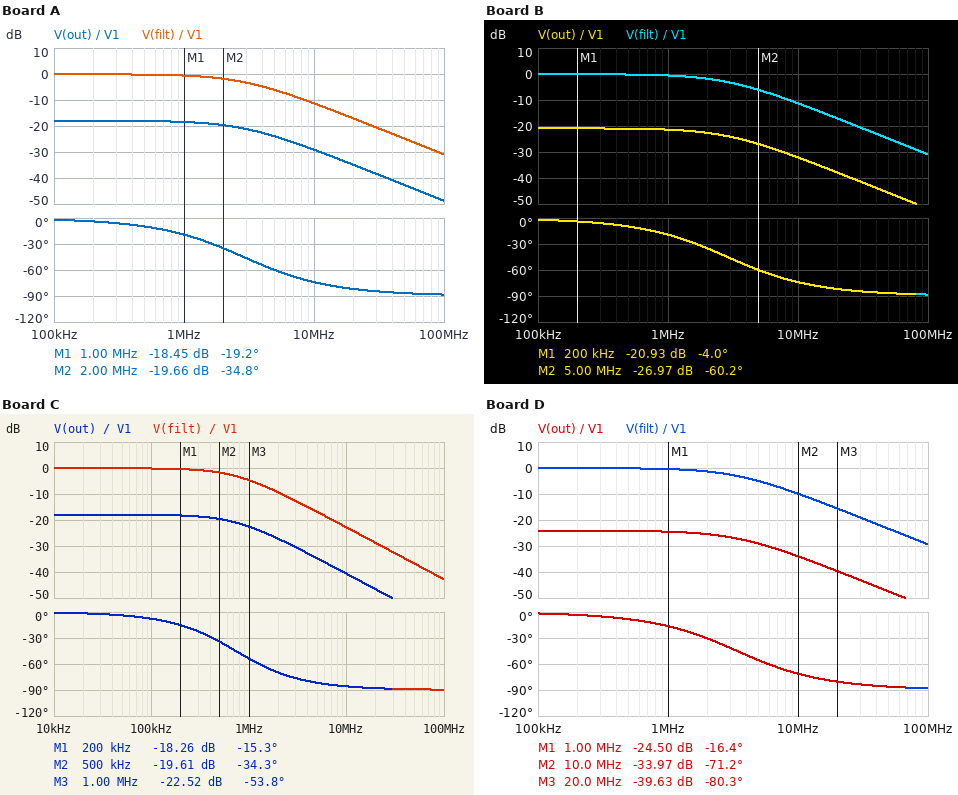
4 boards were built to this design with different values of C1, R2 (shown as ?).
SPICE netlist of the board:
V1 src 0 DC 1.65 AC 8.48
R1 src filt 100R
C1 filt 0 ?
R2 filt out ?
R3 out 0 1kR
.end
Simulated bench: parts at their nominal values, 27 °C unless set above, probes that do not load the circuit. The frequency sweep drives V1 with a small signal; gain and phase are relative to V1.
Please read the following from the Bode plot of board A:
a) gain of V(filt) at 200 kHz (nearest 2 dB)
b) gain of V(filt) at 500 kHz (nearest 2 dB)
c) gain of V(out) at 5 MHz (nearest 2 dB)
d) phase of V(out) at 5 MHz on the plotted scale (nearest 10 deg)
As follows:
0 dB
0 dB
-24 dB
-60 deg
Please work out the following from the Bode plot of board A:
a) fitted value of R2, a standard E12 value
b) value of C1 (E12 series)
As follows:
6.8 kΩ
560 pF
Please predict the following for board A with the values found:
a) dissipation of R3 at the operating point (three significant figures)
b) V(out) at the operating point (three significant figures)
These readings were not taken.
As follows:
43.6 µW
209 mV
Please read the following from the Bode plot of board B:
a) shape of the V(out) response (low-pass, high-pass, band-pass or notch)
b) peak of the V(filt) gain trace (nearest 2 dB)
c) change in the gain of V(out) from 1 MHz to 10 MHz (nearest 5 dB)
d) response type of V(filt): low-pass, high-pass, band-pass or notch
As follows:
low-pass
0 dB
-10 dB
low-pass
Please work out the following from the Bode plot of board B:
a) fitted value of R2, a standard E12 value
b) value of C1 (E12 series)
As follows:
10 kΩ
560 pF
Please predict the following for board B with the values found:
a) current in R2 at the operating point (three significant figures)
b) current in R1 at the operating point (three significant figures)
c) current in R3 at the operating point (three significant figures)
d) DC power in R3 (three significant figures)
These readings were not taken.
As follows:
149 µA
149 µA
149 µA
22.1 µW
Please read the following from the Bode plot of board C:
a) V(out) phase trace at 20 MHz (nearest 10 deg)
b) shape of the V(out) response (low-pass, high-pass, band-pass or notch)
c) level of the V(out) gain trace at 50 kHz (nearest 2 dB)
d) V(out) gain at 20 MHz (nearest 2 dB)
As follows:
-90 deg
low-pass
-18 dB
-46 dB
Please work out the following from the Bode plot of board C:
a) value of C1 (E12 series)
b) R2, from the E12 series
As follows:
2.2 nF
6.8 kΩ
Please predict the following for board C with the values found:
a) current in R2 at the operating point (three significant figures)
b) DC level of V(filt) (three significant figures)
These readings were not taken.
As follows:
209 µA
1.63 V
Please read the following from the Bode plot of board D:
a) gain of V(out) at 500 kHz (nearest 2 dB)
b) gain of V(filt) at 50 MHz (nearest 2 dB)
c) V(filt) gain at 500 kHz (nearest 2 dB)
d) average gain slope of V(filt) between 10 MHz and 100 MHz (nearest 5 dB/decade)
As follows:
-24 dB
-24 dB
0 dB
-20 dB/decade
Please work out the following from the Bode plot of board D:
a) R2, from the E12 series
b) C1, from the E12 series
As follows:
15 kΩ
470 pF
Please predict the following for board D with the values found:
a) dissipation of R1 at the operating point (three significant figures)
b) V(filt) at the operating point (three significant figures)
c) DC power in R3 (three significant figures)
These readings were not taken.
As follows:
1.05 µW
1.64 V
10.5 µW
